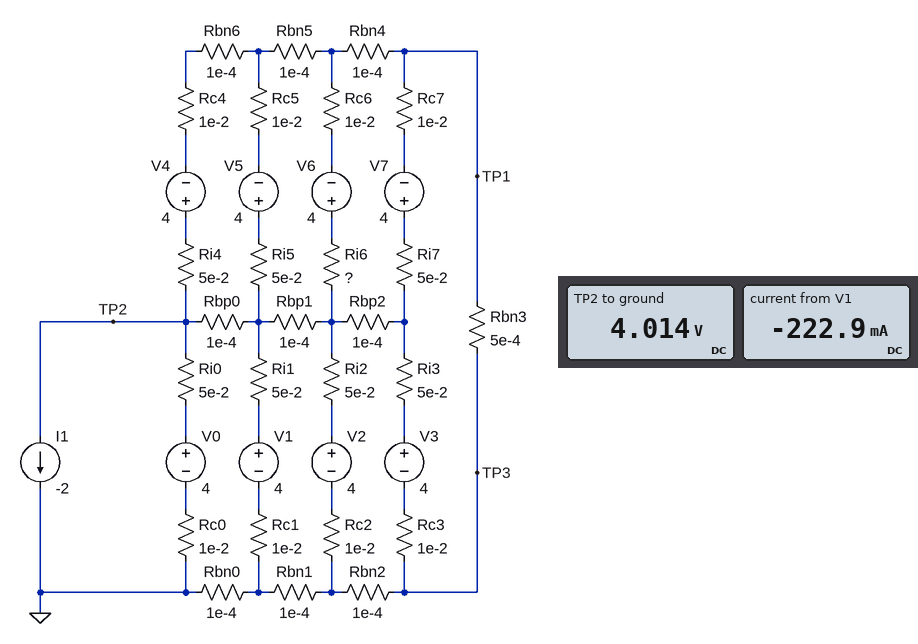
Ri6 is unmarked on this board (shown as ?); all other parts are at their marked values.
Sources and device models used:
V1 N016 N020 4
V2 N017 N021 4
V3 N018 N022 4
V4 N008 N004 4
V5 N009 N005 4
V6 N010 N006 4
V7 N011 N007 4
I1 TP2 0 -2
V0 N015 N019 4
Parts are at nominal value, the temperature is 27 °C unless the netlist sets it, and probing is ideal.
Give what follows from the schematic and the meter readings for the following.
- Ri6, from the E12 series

0.015 Ω
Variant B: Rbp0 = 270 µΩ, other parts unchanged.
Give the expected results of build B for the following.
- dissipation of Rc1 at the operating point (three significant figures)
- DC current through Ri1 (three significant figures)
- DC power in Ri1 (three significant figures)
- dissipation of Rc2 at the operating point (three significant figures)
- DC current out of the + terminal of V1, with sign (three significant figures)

493 µW
222 mA
2.46 mW
473 µW
-222 mA
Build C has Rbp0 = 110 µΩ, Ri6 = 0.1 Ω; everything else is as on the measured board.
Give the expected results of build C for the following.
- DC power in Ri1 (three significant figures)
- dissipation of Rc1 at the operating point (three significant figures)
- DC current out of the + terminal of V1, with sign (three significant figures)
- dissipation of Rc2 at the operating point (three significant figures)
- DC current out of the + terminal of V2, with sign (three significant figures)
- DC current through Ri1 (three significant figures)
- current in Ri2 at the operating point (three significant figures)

3.70 mW
741 µW
-272 mA
719 µW
-268 mA
272 mA
268 mA
